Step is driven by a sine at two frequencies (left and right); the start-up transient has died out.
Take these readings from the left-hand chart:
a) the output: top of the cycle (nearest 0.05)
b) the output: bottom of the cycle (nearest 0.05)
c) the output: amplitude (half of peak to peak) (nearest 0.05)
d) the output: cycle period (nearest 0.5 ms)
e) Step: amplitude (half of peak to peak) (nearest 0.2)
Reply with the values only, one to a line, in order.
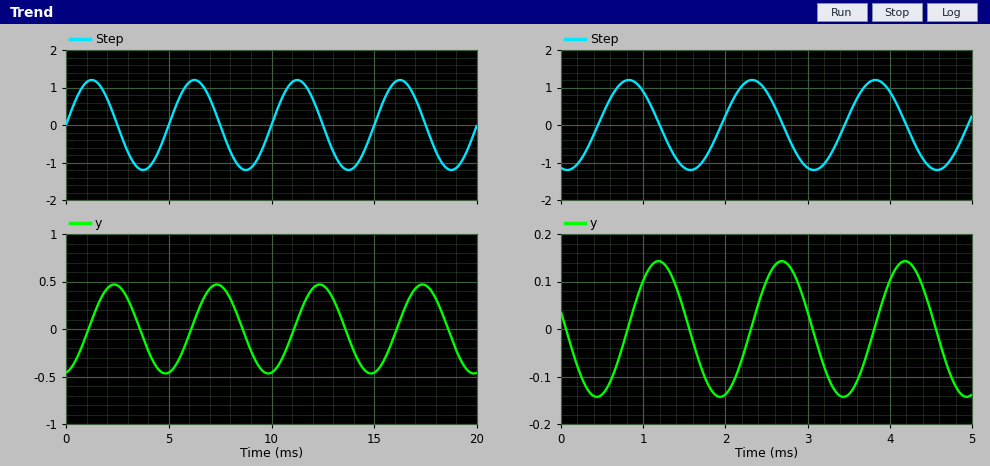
0.45
-0.45
0.45
5.0 ms
1.2
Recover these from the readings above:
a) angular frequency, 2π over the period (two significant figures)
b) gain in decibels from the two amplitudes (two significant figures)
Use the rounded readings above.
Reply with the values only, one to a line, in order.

1.3 rad/ms
-8.5 dB
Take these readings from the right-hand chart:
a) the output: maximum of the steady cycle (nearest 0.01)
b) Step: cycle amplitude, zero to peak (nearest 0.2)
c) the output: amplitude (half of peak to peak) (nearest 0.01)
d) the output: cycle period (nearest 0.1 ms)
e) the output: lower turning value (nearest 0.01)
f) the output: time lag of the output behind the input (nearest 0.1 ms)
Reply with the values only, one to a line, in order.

0.14
1.2
0.14
1.5 ms
-0.14
0.4 ms
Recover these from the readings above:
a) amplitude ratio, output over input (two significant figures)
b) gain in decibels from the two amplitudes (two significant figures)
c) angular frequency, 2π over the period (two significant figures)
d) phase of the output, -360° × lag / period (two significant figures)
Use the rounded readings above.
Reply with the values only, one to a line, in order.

0.12
-19 dB
4.2 rad/ms
-96°
